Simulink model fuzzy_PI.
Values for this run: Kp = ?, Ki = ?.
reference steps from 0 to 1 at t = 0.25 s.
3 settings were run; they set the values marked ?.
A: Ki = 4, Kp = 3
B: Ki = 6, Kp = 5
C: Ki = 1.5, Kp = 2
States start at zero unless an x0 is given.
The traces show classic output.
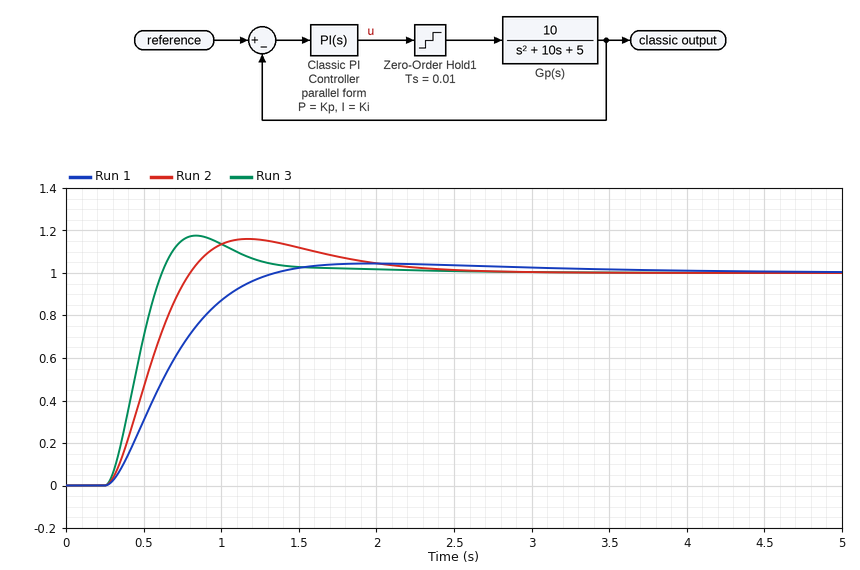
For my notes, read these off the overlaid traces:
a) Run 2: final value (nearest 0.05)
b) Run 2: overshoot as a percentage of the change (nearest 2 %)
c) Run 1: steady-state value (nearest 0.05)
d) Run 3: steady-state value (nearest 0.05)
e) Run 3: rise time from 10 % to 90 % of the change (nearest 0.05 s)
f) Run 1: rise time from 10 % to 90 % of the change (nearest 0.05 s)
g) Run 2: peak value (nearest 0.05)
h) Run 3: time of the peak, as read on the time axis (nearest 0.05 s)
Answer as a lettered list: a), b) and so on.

a) 1.00
b) 16 %
c) 1.00
d) 1.00
e) 0.25 s
f) 0.70 s
g) 1.15
h) 0.85 s
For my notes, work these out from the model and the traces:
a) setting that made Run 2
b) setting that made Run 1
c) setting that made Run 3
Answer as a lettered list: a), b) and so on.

a) A
b) C
c) B
